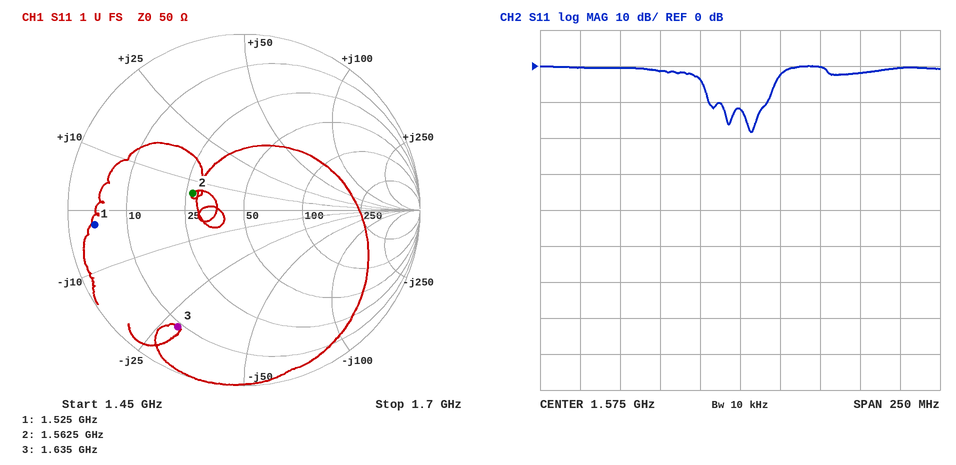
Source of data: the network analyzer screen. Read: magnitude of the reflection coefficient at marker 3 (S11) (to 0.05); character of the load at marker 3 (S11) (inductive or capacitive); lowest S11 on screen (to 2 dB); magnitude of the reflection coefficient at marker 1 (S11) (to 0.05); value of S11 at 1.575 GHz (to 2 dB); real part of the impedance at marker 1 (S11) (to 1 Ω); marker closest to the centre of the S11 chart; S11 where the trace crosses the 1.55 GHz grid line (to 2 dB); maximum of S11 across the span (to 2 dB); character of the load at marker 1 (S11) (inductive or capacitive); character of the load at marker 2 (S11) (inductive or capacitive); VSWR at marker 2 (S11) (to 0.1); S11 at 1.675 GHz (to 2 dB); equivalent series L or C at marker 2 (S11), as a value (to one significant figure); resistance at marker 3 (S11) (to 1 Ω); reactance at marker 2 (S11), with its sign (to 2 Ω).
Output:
0.75
capacitive
-18 dB
0.85
-12 dB
4 Ω
marker 2
-4 dB
0 dB
capacitive
inductive
1.9
0 dB
600 pH
9 Ω
+6 Ω
